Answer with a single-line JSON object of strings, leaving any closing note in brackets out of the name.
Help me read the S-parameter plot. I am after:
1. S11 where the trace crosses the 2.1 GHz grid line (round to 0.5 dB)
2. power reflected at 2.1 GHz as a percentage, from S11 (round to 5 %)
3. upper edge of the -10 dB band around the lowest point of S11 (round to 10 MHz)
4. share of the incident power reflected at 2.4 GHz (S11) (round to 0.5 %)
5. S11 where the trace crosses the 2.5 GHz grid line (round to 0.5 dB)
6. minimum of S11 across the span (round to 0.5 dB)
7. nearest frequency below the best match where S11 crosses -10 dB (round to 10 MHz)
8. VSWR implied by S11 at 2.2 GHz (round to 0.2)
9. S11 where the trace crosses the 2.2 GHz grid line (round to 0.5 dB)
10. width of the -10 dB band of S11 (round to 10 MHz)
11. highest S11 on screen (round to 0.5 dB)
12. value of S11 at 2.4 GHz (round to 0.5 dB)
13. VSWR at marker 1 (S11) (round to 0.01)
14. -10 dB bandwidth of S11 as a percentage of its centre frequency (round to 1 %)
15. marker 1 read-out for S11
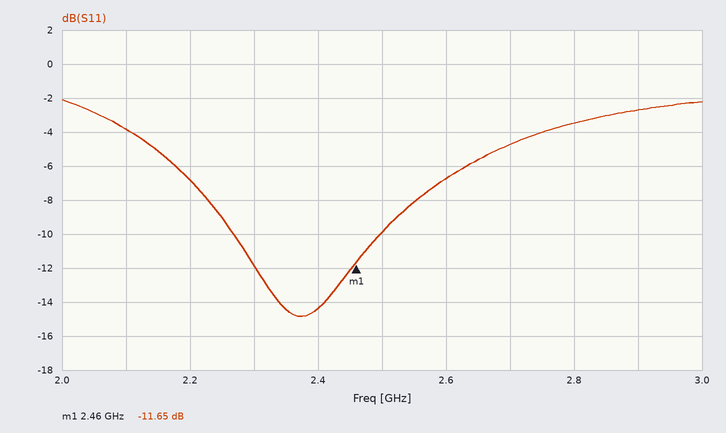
{"S11 where the trace crosses the 2.1 GHz grid line": "-4.0 dB", "power reflected at 2.1 GHz as a percentage, from S11": "40 %", "upper edge of the -10 dB band around the lowest point of S11": "2.50 GHz", "share of the incident power reflected at 2.4 GHz (S11)": "3.5 %", "S11 where the trace crosses the 2.5 GHz grid line": "-10.0 dB", "minimum of S11 across the span": "-15.0 dB", "nearest frequency below the best match where S11 crosses -10 dB": "2.27 GHz", "VSWR implied by S11 at 2.2 GHz": "2.6", "S11 where the trace crosses the 2.2 GHz grid line": "-7.0 dB", "width of the -10 dB band of S11": "230 MHz", "highest S11 on screen": "-2.0 dB", "value of S11 at 2.4 GHz": "-14.5 dB", "VSWR at marker 1 (S11)": "1.71", "-10 dB bandwidth of S11 as a percentage of its centre frequency": "10 %", "marker 1 read-out for S11": "-11.65 dB"}
